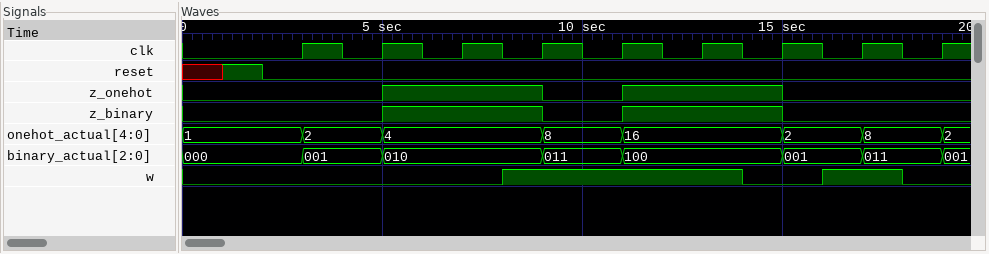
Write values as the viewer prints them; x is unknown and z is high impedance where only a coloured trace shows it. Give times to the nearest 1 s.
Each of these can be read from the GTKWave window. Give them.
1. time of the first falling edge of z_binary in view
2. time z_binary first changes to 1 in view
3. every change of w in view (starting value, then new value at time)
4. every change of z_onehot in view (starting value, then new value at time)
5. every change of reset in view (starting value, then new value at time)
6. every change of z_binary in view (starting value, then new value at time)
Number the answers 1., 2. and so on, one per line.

1. 9 s
2. 5 s
3. 0, 1 at 8 s, 0 at 14 s, 1 at 16 s, 0 at 18 s
4. 0, 1 at 5 s, 0 at 9 s, 1 at 11 s, 0 at 15 s
5. x, 1 at 1 s, 0 at 2 s
6. 0, 1 at 5 s, 0 at 9 s, 1 at 11 s, 0 at 15 s
